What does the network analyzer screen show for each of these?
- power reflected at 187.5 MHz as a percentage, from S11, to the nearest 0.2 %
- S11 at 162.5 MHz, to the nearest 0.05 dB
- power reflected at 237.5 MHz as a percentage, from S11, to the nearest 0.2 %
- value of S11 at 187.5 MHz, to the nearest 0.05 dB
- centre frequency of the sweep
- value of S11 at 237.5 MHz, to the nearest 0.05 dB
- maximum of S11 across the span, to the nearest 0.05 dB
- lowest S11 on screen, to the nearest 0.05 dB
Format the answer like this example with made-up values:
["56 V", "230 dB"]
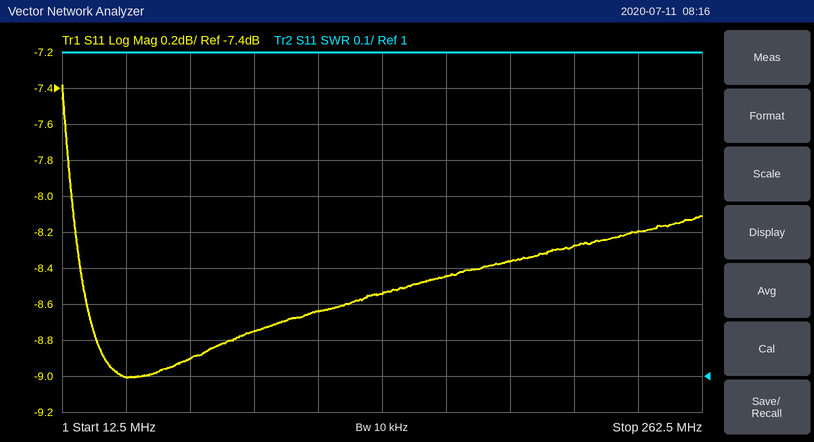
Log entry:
["14.6 %", "-8.45 dB", "15.2 %", "-8.35 dB", "137.5 MHz", "-8.20 dB", "-7.40 dB", "-9.00 dB"]
